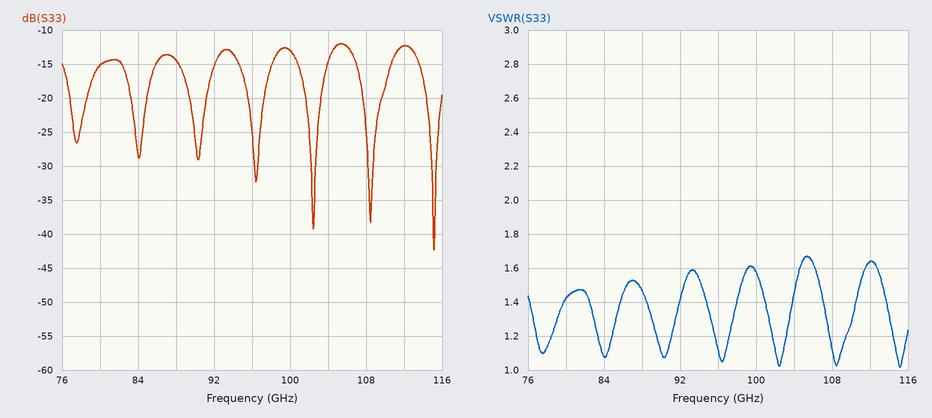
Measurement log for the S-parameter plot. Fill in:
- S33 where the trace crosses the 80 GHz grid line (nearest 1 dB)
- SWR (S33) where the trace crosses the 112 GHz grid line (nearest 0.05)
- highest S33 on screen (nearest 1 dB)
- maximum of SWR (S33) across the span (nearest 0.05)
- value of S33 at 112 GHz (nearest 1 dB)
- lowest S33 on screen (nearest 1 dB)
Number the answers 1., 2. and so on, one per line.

1. -15 dB
2. 1.65
3. -12 dB
4. 1.65
5. -12 dB
6. -42 dB
